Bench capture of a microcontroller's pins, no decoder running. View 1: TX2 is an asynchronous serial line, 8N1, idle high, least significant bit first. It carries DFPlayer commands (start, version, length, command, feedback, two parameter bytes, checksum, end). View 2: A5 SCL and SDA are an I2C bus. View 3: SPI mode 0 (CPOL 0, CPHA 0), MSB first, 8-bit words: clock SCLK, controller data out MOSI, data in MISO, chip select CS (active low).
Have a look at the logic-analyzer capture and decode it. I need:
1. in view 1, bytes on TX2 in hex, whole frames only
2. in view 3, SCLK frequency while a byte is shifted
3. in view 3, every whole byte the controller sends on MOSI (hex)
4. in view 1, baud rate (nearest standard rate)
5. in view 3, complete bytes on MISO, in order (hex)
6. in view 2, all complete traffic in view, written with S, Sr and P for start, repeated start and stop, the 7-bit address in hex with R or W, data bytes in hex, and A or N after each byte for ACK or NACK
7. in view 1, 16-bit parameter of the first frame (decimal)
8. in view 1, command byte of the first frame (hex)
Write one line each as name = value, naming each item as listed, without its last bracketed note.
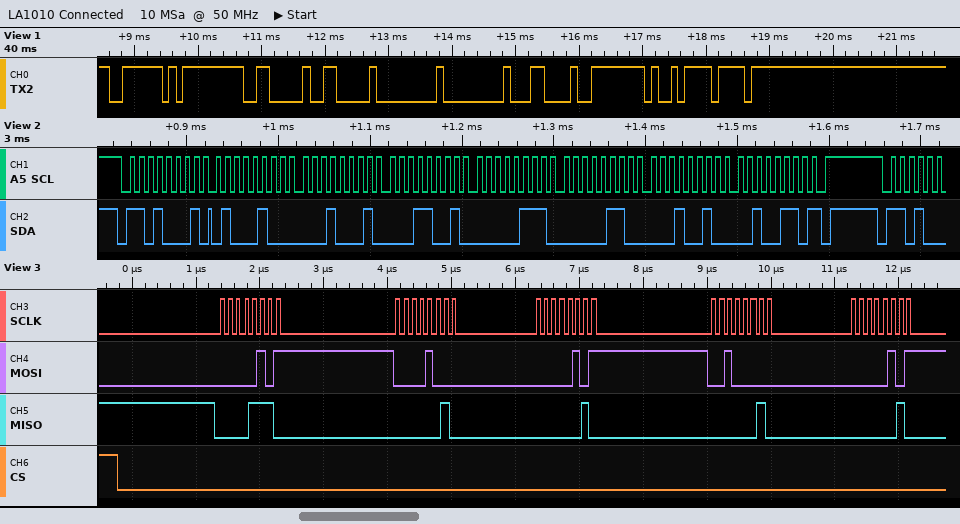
in view 1, bytes on TX2 in hex, whole frames only = 7E FF 06 06 00 00 0C FE E9 EF
in view 3, SCLK frequency while a byte is shifted = 8 MHz
in view 3, every whole byte the controller sends on MOSI = 05 08 05 20 05
in view 1, baud rate = 9600 baud
in view 3, complete bytes on MISO, in order = 0E 02 02 02 02
in view 2, all complete traffic in view, written with S, Sr and P for start, repeated start and stop, the 7-bit address in hex with R or W, data bytes in hex, and A or N after each byte for ACK or NACK = S 68R A 44 A 11 A 19 A 07 A 06 A 12 A 26 N P
in view 1, 16-bit parameter of the first frame = 12
in view 1, command byte of the first frame = 0x06
